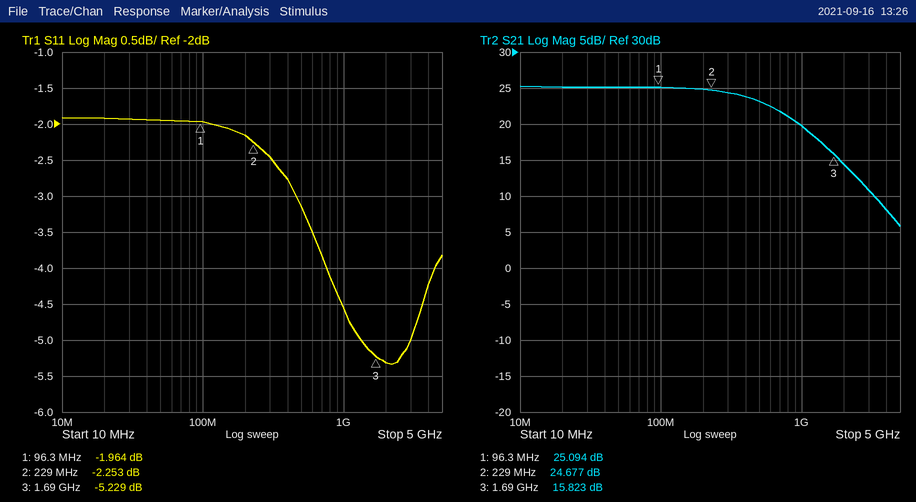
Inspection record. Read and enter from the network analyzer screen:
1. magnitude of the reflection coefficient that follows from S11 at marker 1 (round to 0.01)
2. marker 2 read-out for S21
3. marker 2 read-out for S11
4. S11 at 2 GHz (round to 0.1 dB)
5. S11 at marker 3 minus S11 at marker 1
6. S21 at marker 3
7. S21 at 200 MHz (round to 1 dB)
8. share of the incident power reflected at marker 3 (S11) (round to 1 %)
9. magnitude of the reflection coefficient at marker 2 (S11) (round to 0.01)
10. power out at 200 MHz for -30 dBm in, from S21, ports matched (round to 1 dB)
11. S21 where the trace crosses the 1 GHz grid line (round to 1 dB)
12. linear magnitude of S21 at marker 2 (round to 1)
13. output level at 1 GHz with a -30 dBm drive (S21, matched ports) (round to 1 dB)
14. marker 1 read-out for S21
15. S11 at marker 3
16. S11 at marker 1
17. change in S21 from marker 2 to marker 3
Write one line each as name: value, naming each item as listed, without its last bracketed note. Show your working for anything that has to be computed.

magnitude of the reflection coefficient that follows from S11 at marker 1: 10^(-1.964/20) ≈ 0.80
marker 2 read-out for S21: 24.677 dB
marker 2 read-out for S11: -2.253 dB
S11 at 2 GHz: -5.3 dB
S11 at marker 3 minus S11 at marker 1: -5.229 − (-1.964) = -3.265 dB
S21 at marker 3: 15.823 dB
S21 at 200 MHz: 25 dB
share of the incident power reflected at marker 3 (S11): 10^(-5.229/10) ≈ 30 %
magnitude of the reflection coefficient at marker 2 (S11): 10^(-2.253/20) ≈ 0.77
power out at 200 MHz for -30 dBm in, from S21, ports matched: -30 dBm + (25 dB) = -5 dBm
S21 where the trace crosses the 1 GHz grid line: 20 dB
linear magnitude of S21 at marker 2: 10^(24.677/20) ≈ 17
output level at 1 GHz with a -30 dBm drive (S21, matched ports): -30 dBm + (20 dB) = -10 dBm
marker 1 read-out for S21: 25.094 dB
S11 at marker 3: -5.229 dB
S11 at marker 1: -1.964 dB
change in S21 from marker 2 to marker 3: 15.823 − (24.677) = -8.854 dB
